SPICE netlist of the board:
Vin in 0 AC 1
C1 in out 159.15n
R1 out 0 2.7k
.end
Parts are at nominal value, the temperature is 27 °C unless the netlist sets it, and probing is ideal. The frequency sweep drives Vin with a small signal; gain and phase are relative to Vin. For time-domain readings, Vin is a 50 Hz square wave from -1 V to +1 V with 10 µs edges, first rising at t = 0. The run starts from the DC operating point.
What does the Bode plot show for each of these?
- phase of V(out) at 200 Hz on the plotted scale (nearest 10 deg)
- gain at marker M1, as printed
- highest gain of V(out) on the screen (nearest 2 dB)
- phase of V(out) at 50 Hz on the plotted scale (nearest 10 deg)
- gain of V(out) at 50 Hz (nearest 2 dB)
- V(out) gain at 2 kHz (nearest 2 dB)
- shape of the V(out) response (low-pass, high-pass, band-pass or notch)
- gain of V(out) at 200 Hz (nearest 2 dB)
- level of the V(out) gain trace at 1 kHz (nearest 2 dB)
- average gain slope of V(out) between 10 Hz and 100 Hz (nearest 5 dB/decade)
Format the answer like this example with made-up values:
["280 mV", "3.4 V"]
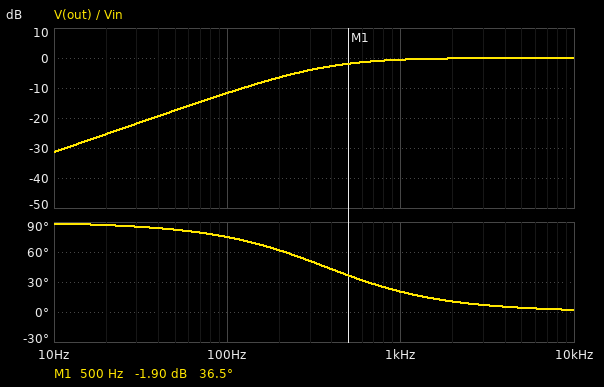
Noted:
["60 deg", "-1.90 dB", "0 dB", "80 deg", "-18 dB", "0 dB", "high-pass", "-6 dB", "0 dB", "20 dB/decade"]
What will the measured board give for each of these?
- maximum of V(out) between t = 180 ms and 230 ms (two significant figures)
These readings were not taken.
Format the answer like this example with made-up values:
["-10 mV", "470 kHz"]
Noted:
["2.0 V"]
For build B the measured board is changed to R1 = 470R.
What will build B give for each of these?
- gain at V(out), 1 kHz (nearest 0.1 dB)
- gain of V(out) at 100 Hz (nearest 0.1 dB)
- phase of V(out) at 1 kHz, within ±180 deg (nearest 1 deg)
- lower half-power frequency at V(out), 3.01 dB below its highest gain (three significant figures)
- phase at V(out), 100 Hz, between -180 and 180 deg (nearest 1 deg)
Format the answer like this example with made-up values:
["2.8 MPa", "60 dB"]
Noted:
["-7.4 dB", "-26.6 dB", "65 deg", "2.13 kHz", "87 deg"]
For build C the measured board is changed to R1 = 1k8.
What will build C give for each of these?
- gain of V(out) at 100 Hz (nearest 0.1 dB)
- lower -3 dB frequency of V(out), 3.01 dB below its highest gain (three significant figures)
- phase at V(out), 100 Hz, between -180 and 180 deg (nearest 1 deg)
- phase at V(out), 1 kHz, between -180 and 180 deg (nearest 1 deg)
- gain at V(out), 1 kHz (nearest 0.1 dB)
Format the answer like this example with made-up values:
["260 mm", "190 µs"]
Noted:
["-15.0 dB", "556 Hz", "80 deg", "29 deg", "-1.2 dB"]
